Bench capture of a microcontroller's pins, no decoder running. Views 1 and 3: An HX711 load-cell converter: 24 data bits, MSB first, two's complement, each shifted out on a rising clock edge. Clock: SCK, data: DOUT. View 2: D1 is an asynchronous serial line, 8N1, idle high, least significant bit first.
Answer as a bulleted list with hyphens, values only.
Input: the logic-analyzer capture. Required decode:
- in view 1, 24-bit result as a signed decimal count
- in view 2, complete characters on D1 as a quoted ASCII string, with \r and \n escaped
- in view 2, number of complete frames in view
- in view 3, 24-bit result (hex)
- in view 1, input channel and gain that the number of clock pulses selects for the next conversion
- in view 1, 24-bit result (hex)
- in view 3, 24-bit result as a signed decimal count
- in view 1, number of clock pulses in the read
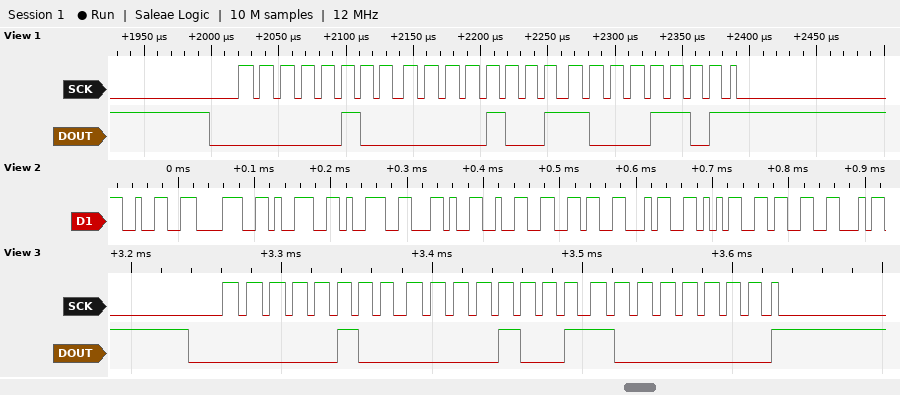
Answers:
- 264589
- "2899,26453"
- 10
- 0x040980
- channel A, gain 128
- 0x04098D
- 264576
- 25
